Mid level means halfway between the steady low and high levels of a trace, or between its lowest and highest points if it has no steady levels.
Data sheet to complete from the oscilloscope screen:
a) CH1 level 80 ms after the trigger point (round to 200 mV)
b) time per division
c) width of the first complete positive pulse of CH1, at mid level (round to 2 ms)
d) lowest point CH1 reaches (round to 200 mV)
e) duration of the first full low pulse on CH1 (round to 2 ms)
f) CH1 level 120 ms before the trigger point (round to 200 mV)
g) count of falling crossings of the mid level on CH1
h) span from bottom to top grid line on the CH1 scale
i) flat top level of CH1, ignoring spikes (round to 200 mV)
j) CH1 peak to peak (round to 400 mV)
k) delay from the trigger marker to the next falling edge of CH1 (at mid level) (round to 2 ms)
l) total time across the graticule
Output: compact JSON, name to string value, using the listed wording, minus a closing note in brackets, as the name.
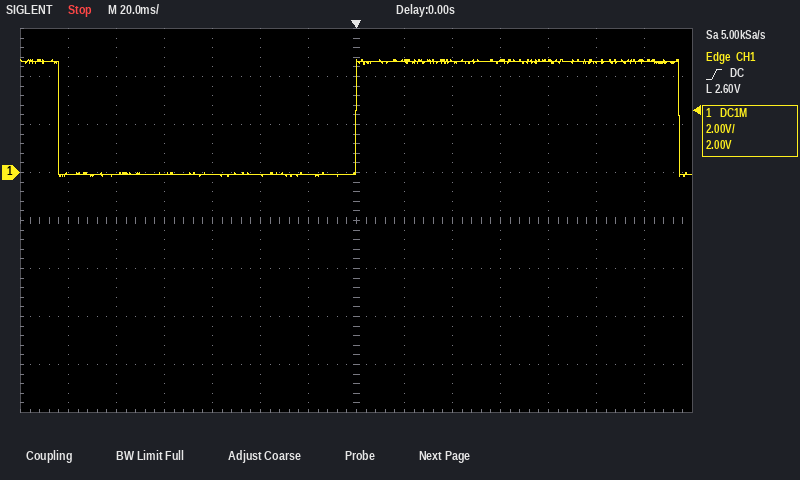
{"CH1 level 80 ms after the trigger point": "4.6 V", "time per division": "20 ms", "width of the first complete positive pulse of CH1, at mid level": "134 ms", "lowest point CH1 reaches": "-200 mV", "duration of the first full low pulse on CH1": "124 ms", "CH1 level 120 ms before the trigger point": "0.0 V", "count of falling crossings of the mid level on CH1": "2", "span from bottom to top grid line on the CH1 scale": "16 V", "flat top level of CH1, ignoring spikes": "4.6 V", "CH1 peak to peak": "4.8 V", "delay from the trigger marker to the next falling edge of CH1 (at mid level)": "134 ms", "total time across the graticule": "280 ms"}
